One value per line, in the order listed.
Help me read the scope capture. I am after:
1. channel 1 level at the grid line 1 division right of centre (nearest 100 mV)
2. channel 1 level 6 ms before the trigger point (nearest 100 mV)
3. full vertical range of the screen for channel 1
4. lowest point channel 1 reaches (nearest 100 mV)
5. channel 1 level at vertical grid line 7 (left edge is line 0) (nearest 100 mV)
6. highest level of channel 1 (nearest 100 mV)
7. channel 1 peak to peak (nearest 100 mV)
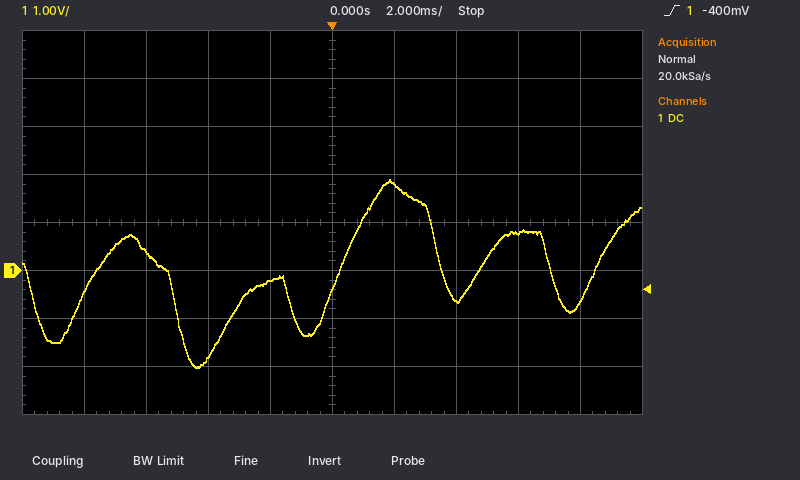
1.8 V
400 mV
8 V
-2.0 V
-600 mV
1.9 V
3.9 V
